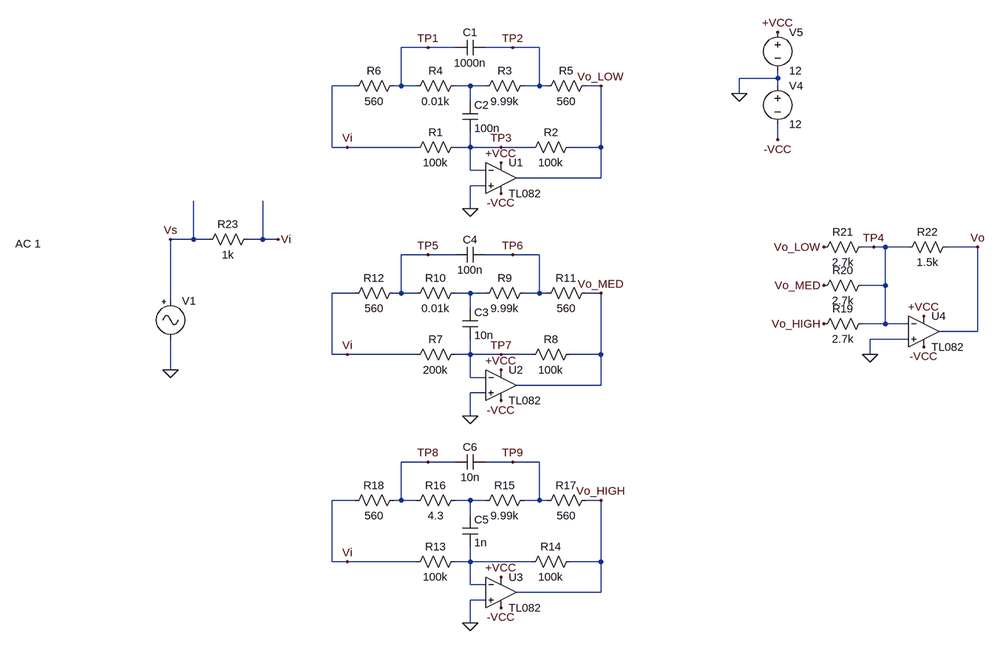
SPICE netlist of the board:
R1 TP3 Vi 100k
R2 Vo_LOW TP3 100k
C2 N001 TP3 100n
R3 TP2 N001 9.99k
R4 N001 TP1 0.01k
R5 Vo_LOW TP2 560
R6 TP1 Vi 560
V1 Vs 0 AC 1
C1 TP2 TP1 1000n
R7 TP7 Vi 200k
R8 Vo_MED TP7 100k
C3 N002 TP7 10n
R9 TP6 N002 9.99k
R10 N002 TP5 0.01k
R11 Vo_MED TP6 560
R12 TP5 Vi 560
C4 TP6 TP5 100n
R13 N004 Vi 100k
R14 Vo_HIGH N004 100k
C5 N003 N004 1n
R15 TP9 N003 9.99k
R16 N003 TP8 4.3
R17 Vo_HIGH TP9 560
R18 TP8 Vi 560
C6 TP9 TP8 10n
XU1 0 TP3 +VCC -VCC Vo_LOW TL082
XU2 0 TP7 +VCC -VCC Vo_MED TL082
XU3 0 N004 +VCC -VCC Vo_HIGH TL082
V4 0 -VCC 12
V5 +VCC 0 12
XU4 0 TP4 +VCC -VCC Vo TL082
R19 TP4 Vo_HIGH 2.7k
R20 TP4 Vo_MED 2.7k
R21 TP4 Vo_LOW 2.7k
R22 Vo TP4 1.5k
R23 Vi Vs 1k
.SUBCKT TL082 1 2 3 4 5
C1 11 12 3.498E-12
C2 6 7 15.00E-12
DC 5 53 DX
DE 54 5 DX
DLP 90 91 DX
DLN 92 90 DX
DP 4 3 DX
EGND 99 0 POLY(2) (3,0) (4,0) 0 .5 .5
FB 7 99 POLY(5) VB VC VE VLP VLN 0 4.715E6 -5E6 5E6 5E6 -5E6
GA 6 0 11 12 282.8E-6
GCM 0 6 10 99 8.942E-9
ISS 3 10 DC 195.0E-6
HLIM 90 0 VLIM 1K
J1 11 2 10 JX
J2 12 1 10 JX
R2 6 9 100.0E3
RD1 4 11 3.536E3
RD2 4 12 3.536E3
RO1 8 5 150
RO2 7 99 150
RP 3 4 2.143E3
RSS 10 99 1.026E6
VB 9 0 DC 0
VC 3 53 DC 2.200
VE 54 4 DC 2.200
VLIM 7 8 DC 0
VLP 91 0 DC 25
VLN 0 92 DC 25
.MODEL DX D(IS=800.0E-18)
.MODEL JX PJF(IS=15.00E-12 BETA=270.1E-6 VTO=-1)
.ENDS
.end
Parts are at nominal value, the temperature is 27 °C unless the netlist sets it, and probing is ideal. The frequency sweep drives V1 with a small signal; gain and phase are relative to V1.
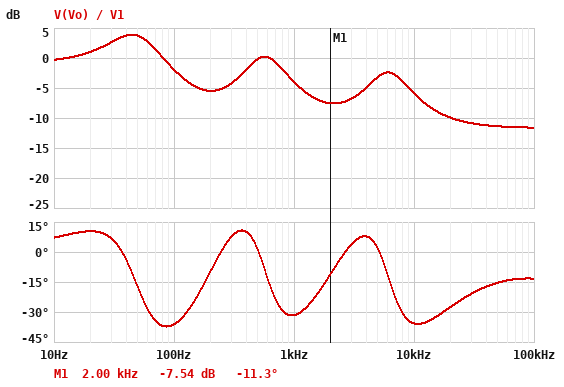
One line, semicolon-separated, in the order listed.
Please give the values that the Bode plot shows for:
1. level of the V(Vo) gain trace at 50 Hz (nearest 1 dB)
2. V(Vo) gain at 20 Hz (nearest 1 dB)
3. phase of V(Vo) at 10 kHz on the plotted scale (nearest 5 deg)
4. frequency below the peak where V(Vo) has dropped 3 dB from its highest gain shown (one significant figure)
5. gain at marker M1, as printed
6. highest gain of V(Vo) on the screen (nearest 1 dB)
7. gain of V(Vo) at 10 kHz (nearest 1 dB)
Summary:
4 dB; 1 dB; -35 deg; 20 Hz; -7.54 dB; 4 dB; -6 dB
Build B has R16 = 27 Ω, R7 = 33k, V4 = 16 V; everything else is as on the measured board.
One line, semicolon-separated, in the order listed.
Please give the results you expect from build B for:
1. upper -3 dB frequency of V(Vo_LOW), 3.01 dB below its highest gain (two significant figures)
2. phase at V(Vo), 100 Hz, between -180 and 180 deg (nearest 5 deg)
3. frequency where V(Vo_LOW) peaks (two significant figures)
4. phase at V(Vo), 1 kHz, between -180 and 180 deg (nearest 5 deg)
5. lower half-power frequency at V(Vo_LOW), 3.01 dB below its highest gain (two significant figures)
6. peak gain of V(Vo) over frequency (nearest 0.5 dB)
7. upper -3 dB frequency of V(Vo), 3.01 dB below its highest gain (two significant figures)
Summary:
82 Hz; -30 deg; 50 Hz; -40 deg; 30 Hz; 6.0 dB; 72 Hz
